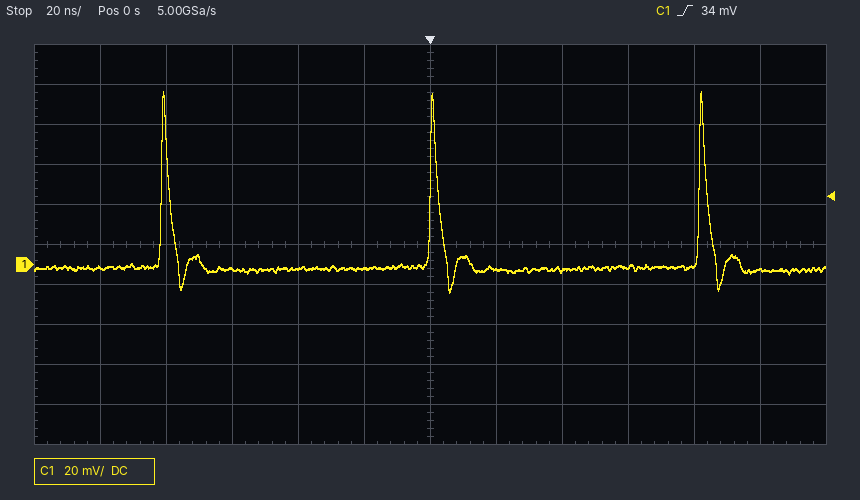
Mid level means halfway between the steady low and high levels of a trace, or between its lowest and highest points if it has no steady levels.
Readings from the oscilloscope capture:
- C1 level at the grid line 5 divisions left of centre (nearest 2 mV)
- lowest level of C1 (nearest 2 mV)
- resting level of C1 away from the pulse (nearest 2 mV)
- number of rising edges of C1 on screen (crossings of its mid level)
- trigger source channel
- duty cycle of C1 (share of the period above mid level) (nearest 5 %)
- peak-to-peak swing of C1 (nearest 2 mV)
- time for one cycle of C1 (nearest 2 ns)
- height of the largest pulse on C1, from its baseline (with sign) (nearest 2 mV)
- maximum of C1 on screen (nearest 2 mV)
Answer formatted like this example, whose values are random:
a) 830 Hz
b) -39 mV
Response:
a) -2 mV
b) -14 mV
c) -2 mV
d) 3
e) C1
f) 5 %
g) 100 mV
h) 82 ns
i) +88 mV
j) 86 mV
